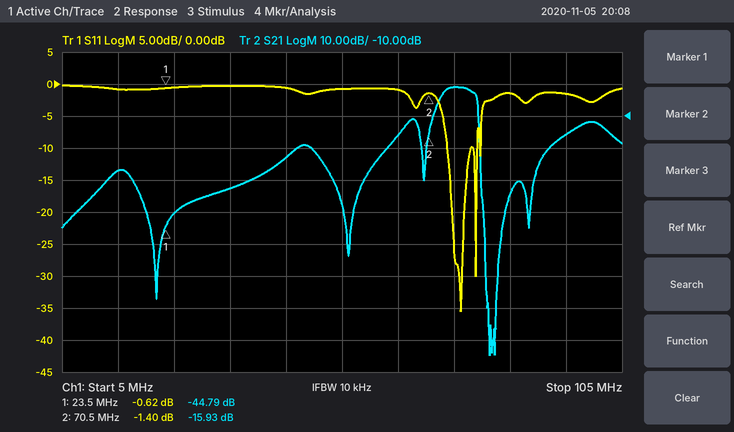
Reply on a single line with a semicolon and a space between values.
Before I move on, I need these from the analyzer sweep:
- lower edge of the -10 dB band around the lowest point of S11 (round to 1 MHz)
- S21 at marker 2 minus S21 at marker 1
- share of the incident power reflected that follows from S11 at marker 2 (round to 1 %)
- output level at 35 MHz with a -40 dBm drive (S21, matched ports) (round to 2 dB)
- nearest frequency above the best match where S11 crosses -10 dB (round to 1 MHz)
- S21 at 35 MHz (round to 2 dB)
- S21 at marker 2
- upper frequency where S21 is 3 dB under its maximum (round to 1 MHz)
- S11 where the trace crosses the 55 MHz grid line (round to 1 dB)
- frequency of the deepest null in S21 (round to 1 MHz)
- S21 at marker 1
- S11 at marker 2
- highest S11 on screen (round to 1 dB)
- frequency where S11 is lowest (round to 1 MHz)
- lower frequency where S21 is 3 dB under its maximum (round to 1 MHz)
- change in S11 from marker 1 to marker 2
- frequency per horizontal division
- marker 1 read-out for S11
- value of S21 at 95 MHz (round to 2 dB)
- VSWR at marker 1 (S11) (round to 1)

74 MHz; 28.86 dB; 72 %; -72 dBm; 78 MHz; -32 dB; -15.93 dB; 79 MHz; -1 dB; 81 MHz; -44.79 dB; -1.40 dB; 0 dB; 76 MHz; 73 MHz; -0.78 dB; 10 MHz; -0.62 dB; -16 dB; 28
